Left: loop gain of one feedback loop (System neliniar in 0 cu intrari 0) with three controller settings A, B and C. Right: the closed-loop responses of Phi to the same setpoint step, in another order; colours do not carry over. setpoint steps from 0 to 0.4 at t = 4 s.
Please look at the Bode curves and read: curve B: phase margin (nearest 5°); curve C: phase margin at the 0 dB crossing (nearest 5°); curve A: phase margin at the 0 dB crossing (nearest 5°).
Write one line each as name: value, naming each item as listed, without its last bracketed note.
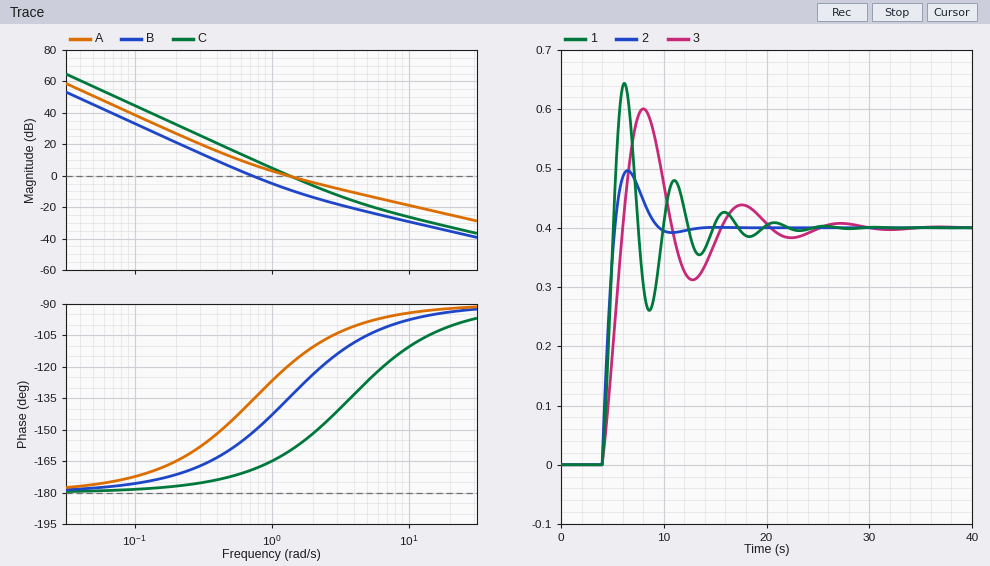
curve B: phase margin: 30°
curve C: phase margin at the 0 dB crossing: 20°
curve A: phase margin at the 0 dB crossing: 60°
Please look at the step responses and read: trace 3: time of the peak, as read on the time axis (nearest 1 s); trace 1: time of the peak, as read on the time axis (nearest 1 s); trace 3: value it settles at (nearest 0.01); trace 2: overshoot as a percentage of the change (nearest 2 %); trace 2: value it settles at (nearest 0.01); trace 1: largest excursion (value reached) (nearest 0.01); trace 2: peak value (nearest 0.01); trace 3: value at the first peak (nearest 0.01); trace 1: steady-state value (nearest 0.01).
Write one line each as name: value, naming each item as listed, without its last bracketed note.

trace 3: time of the peak, as read on the time axis: 8 s
trace 1: time of the peak, as read on the time axis: 6 s
trace 3: value it settles at: 0.40
trace 2: overshoot as a percentage of the change: 24 %
trace 2: value it settles at: 0.40
trace 1: largest excursion (value reached): 0.64
trace 2: peak value: 0.50
trace 3: value at the first peak: 0.60
trace 1: steady-state value: 0.40
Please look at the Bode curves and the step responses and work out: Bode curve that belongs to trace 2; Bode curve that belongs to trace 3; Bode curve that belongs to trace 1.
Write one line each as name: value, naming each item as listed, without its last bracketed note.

Bode curve that belongs to trace 2: A
Bode curve that belongs to trace 3: B
Bode curve that belongs to trace 1: C
